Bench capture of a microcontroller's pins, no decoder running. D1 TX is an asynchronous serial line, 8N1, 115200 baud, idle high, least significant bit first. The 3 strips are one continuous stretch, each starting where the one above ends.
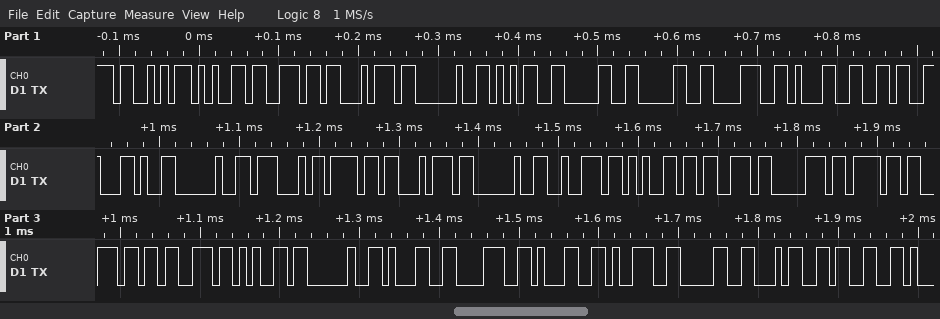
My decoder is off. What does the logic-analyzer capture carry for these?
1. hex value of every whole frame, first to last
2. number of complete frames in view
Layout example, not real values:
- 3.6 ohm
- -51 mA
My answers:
- 53 65 6E 74 20 35 30 30 38 31 36 2C 20 47 6F 74 20 72 65 73 70 6F 6E 73 65 20 31 38 31 39 30 34 33
- 33
